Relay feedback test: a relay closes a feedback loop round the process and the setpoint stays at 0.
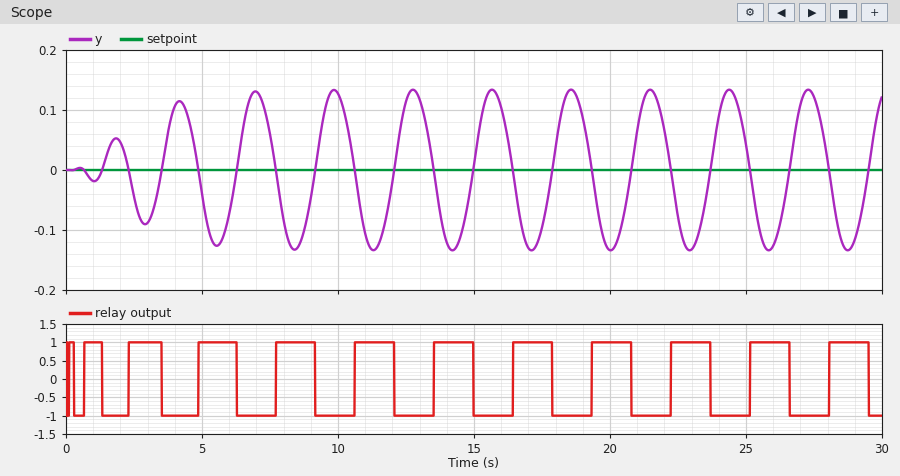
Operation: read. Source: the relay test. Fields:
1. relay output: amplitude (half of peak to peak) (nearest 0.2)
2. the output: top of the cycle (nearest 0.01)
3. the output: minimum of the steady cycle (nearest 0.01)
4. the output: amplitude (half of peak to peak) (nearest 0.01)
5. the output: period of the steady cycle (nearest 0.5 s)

1.0
0.13
-0.13
0.13
3.0 s
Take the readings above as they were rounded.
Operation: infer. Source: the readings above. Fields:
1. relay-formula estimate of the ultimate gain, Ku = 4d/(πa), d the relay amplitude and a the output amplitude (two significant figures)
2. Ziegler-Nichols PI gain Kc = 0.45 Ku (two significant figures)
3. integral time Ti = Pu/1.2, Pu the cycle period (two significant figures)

9.8
4.4
2.5 s
